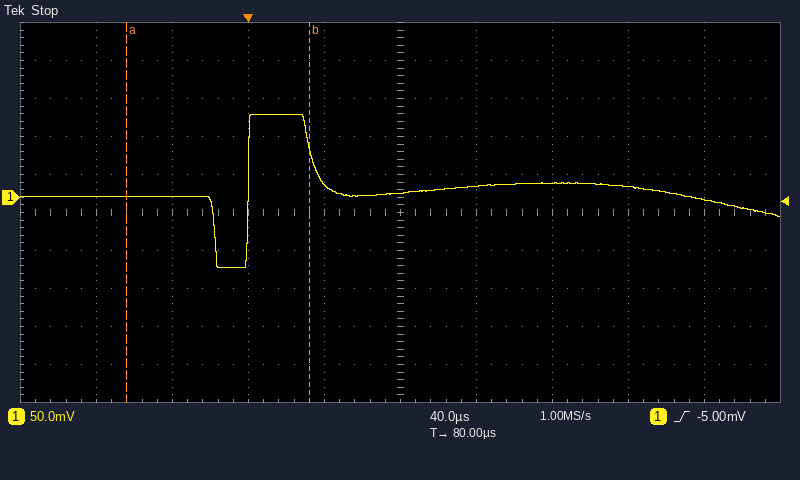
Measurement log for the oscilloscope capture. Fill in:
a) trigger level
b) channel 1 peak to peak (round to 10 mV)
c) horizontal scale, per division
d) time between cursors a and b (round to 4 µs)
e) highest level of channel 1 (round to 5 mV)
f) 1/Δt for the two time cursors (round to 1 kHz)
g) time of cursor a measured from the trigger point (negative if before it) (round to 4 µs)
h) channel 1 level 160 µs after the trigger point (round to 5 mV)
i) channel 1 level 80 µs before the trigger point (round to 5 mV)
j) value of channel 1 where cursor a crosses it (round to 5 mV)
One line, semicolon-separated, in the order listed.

-5.00 mV; 200 mV; 40 µs; 96 µs; 110 mV; 10 kHz; -64 µs; 20 mV; 0 mV; 0 mV
